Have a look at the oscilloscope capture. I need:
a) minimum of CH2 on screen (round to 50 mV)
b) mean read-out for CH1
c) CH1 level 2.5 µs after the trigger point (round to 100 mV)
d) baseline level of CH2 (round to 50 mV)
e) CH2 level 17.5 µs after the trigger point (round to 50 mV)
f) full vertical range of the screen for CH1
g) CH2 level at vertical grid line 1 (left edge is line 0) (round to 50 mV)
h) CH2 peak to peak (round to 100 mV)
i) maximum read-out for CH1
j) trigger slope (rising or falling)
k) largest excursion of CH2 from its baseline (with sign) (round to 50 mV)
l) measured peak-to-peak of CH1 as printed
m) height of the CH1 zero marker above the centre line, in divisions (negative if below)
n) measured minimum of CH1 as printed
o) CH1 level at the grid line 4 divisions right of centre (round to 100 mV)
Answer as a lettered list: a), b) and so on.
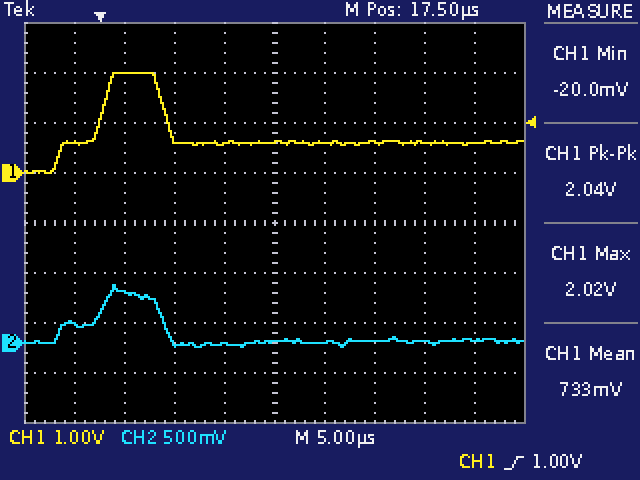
a) -50 mV
b) 733 mV
c) 2.0 V
d) 0 mV
e) 0 mV
f) 8 V
g) 200 mV
h) 600 mV
i) 2.02 V
j) rising
k) +550 mV
l) 2.04 V
m) +1.0 div
n) -20.0 mV
o) 600 mV
